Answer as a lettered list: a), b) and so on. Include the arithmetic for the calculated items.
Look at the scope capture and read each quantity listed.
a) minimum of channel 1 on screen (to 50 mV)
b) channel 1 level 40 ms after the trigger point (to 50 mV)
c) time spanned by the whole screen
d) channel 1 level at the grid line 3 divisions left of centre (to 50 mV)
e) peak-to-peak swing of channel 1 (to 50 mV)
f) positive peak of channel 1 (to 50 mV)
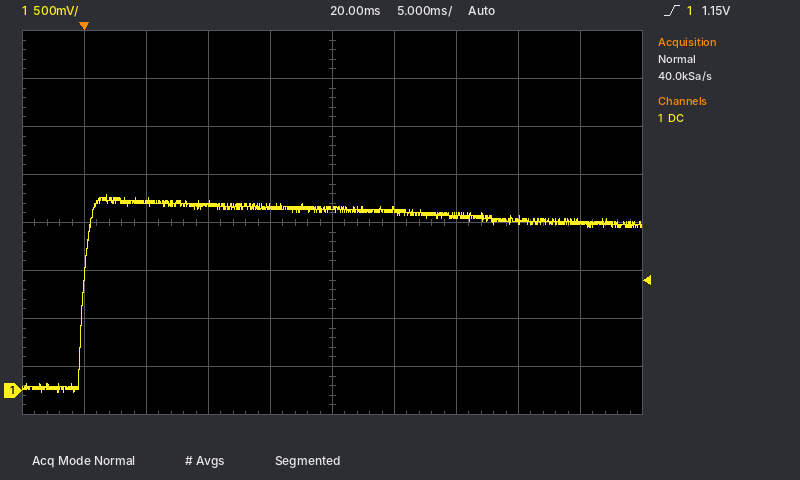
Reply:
a) 0 mV
b) 1.75 V
c) 50 ms
d) 2.00 V
e) 2.05 V − (0 mV) = 2.05 V
f) 2.05 V
